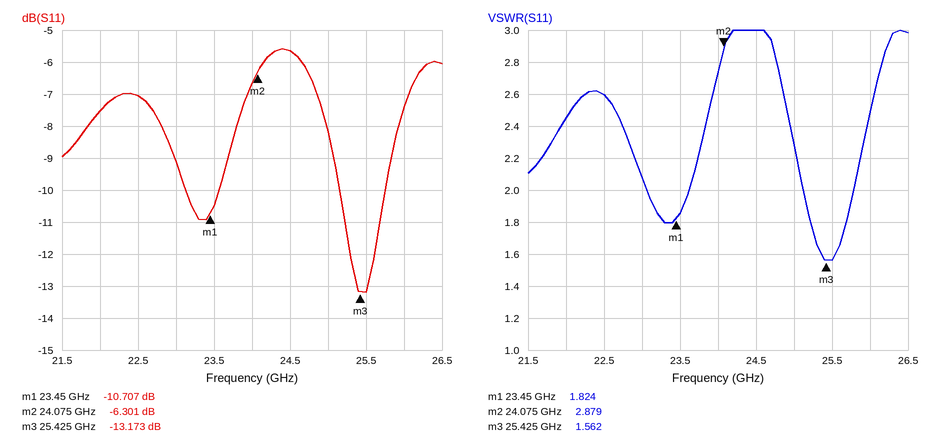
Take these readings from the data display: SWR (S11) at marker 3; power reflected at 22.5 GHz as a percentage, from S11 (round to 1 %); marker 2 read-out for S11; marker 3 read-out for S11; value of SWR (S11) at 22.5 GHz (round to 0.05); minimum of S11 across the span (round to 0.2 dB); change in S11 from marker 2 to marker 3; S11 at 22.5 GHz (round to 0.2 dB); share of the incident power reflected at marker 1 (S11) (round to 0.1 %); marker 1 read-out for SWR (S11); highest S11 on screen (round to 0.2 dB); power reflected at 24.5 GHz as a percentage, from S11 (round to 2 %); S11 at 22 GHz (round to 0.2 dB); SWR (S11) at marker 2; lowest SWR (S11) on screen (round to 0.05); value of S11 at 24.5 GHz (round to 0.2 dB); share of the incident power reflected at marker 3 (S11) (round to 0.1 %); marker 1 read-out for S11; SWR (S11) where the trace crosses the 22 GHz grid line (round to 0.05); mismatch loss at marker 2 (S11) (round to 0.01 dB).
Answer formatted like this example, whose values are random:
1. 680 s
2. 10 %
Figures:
1. 1.562
2. 20 %
3. -6.301 dB
4. -13.173 dB
5. 2.60
6. -13.2 dB
7. -6.872 dB
8. -7.0 dB
9. 8.5 %
10. 1.824
11. -5.6 dB
12. 28 %
13. -7.6 dB
14. 2.879
15. 1.55
16. -5.6 dB
17. 4.8 %
18. -10.707 dB
19. 2.45
20. 1.16 dB
